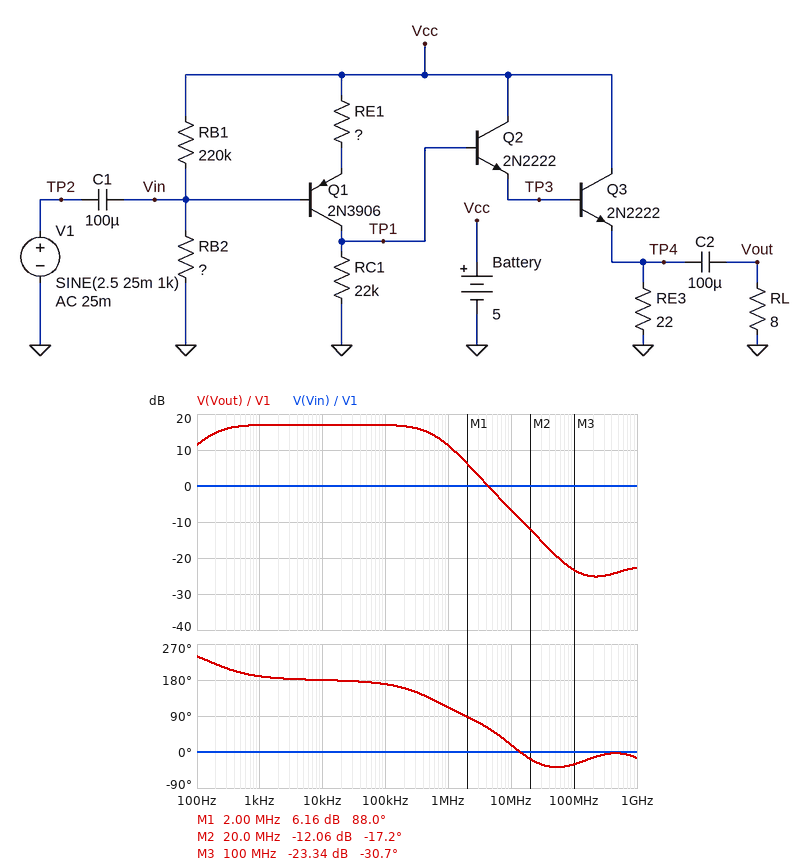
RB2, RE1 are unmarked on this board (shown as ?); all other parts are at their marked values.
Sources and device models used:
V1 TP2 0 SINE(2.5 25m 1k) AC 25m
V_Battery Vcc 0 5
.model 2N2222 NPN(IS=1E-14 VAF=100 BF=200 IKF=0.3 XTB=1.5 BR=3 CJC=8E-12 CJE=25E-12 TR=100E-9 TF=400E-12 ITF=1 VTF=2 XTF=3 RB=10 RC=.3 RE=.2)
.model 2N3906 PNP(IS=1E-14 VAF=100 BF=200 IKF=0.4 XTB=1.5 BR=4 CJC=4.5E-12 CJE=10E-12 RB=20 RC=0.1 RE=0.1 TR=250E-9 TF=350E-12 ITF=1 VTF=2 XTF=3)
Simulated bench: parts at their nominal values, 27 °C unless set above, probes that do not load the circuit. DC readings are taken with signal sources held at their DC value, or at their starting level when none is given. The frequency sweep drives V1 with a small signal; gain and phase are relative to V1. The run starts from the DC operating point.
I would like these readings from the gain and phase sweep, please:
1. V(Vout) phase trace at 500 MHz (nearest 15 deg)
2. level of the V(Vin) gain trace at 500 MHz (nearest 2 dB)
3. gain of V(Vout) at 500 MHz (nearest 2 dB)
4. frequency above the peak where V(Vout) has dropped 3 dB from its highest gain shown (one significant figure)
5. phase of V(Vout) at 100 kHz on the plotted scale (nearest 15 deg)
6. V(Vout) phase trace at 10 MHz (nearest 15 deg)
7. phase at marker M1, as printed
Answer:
0 deg
0 dB
-24 dB
600 kHz
165 deg
15 deg
88.0 deg
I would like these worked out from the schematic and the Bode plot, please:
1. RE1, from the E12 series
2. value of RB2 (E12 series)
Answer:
2.2 kΩ
680 kΩ
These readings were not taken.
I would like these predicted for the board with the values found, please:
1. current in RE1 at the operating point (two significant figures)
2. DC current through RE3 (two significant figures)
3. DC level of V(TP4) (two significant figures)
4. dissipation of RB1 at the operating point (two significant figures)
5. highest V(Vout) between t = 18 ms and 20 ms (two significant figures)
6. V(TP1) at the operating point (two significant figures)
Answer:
200 µA
130 mA
2.8 V
5.1 µW
150 mV
4.3 V
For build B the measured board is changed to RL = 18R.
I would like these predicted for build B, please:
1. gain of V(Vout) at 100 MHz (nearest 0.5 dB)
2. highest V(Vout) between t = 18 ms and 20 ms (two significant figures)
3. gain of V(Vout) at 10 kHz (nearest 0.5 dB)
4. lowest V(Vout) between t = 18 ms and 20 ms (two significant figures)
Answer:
-20.0 dB
160 mV
18.0 dB
-190 mV
